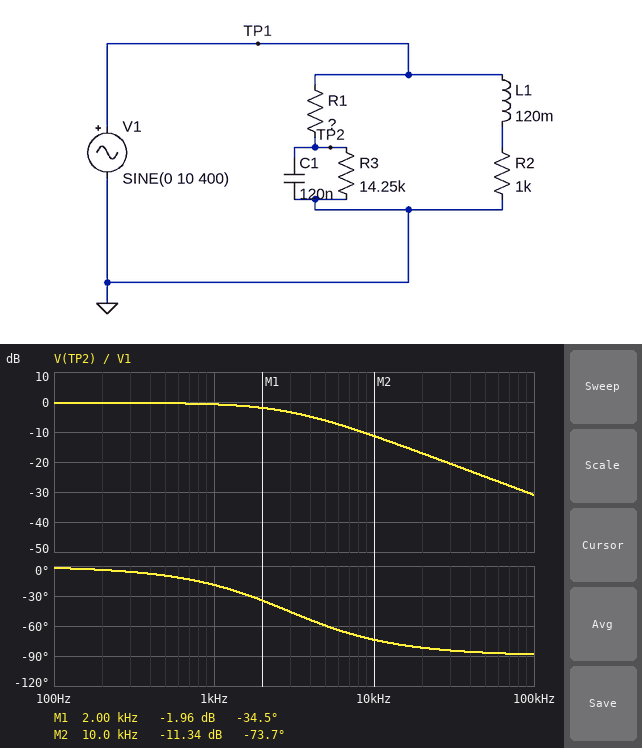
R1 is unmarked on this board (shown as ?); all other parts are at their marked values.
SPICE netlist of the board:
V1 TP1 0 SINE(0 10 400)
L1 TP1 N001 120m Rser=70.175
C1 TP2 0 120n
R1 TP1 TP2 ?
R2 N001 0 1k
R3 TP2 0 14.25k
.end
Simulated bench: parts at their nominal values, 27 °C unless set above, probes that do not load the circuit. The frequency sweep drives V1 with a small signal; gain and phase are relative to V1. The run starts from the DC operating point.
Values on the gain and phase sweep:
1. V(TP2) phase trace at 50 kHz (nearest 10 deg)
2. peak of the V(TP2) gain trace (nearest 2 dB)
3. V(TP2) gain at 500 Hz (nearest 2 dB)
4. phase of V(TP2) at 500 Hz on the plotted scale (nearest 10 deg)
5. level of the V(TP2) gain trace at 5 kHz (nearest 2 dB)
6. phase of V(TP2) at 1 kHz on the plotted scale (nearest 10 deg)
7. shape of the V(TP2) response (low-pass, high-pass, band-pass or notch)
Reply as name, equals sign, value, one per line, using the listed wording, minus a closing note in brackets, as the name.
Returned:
V(TP2) phase trace at 50 kHz = -90 deg
peak of the V(TP2) gain trace = 0 dB
V(TP2) gain at 500 Hz = 0 dB
phase of V(TP2) at 500 Hz on the plotted scale = -10 deg
level of the V(TP2) gain trace at 5 kHz = -6 dB
phase of V(TP2) at 1 kHz on the plotted scale = -20 deg
shape of the V(TP2) response = low-pass
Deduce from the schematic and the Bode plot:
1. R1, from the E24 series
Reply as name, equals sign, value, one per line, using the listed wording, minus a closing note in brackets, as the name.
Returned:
R1, from the E24 series = 470 Ω
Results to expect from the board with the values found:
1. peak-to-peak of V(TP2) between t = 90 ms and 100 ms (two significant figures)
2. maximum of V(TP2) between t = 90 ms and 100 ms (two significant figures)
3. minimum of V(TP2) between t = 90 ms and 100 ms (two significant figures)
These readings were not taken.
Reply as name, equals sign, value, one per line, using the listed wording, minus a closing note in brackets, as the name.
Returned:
peak-to-peak of V(TP2) between t = 90 ms and 100 ms = 19 V
maximum of V(TP2) between t = 90 ms and 100 ms = 9.6 V
minimum of V(TP2) between t = 90 ms and 100 ms = -9.6 V
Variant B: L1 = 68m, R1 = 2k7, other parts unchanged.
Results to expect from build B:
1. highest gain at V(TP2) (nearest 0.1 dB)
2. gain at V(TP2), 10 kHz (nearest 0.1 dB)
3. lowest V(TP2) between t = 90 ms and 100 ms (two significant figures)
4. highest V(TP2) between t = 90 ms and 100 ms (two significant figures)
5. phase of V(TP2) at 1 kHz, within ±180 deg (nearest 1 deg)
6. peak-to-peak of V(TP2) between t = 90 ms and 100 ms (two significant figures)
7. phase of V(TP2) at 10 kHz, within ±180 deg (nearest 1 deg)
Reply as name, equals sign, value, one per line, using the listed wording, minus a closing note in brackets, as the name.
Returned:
highest gain at V(TP2) = -1.5 dB
gain at V(TP2), 10 kHz = -26.2 dB
lowest V(TP2) between t = 90 ms and 100 ms = -6.9 V
highest V(TP2) between t = 90 ms and 100 ms = 6.9 V
phase of V(TP2) at 1 kHz, within ±180 deg = -60 deg
peak-to-peak of V(TP2) between t = 90 ms and 100 ms = 14 V
phase of V(TP2) at 10 kHz, within ±180 deg = -87 deg
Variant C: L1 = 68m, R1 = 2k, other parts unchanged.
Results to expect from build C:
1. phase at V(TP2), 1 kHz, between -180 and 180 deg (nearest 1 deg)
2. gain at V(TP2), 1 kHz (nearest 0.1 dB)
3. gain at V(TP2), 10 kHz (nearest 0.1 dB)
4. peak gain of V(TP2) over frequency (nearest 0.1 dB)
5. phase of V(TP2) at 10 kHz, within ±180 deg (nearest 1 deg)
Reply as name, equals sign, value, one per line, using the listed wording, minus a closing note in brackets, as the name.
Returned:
phase at V(TP2), 1 kHz, between -180 and 180 deg = -53 deg
gain at V(TP2), 1 kHz = -5.5 dB
gain at V(TP2), 10 kHz = -23.6 dB
peak gain of V(TP2) over frequency = -1.1 dB
phase of V(TP2) at 10 kHz, within ±180 deg = -86 deg
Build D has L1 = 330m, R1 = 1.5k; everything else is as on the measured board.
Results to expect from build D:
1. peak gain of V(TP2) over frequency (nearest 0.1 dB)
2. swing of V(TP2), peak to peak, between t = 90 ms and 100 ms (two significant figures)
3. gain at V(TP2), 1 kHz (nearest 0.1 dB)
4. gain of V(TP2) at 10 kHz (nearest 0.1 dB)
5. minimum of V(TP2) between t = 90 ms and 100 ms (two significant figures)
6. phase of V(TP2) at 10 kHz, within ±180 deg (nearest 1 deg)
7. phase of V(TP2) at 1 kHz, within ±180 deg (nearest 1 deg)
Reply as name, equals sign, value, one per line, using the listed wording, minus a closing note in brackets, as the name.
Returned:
peak gain of V(TP2) over frequency = -0.9 dB
swing of V(TP2), peak to peak, between t = 90 ms and 100 ms = 17 V
gain at V(TP2), 1 kHz = -4.0 dB
gain of V(TP2) at 10 kHz = -21.1 dB
minimum of V(TP2) between t = 90 ms and 100 ms = -8.4 V
phase of V(TP2) at 10 kHz, within ±180 deg = -84 deg
phase of V(TP2) at 1 kHz, within ±180 deg = -46 deg
